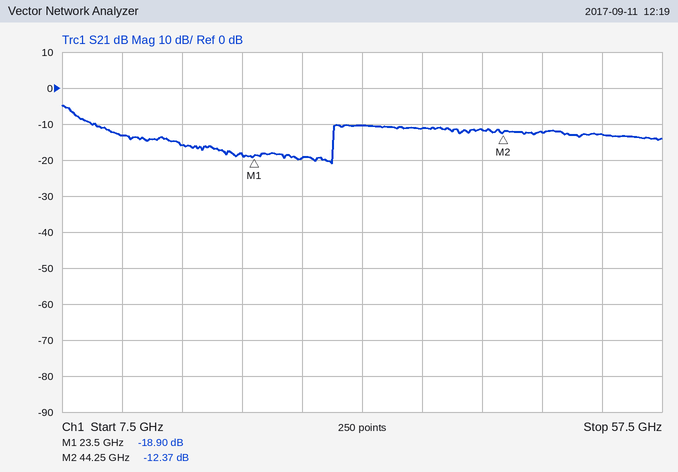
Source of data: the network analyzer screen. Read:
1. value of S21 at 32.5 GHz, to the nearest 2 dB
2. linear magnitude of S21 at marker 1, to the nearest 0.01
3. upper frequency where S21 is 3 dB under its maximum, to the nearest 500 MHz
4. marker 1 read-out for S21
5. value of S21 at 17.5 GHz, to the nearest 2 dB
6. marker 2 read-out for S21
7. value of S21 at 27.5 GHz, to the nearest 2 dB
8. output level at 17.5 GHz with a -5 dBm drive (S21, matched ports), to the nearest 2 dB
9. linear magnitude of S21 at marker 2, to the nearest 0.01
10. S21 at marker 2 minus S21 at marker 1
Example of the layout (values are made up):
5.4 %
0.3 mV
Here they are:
-10 dB
0.11
9.0 GHz
-18.90 dB
-16 dB
-12.37 dB
-20 dB
-20 dBm
0.24
6.53 dB
